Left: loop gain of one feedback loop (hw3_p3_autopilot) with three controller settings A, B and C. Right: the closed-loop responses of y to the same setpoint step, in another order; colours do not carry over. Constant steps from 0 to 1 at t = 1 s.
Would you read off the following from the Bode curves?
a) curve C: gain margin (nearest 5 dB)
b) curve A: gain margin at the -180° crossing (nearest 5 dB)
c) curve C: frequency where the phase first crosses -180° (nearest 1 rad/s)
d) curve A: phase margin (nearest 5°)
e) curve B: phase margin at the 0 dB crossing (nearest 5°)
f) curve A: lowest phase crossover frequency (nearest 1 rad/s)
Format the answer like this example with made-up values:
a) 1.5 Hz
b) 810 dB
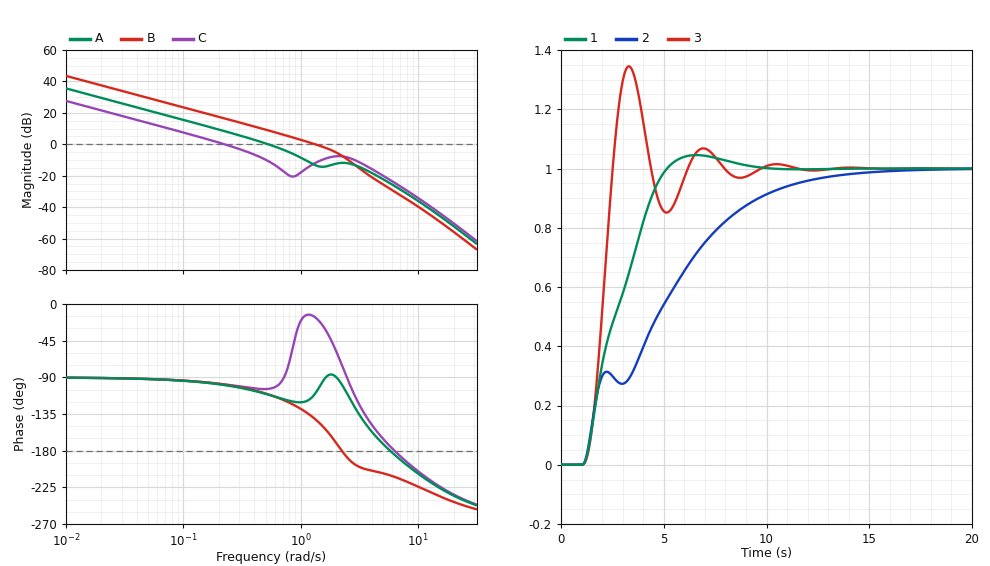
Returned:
a) 25 dB
b) 25 dB
c) 6 rad/s
d) 70°
e) 40°
f) 6 rad/s
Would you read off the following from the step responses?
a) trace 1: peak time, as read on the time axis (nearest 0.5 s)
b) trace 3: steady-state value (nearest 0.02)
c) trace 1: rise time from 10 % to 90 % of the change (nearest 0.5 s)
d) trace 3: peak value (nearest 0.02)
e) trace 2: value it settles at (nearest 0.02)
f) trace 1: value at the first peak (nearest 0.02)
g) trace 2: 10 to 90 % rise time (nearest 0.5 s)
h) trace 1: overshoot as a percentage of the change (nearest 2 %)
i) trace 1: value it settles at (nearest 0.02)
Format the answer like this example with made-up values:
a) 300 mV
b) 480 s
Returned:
a) 6.5 s
b) 1.00
c) 3.0 s
d) 1.34
e) 1.00
f) 1.04
g) 8.0 s
h) 4 %
i) 1.00
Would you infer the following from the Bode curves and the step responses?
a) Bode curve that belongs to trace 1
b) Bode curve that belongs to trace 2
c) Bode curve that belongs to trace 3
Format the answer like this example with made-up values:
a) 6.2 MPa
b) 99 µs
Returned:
a) A
b) C
c) B
